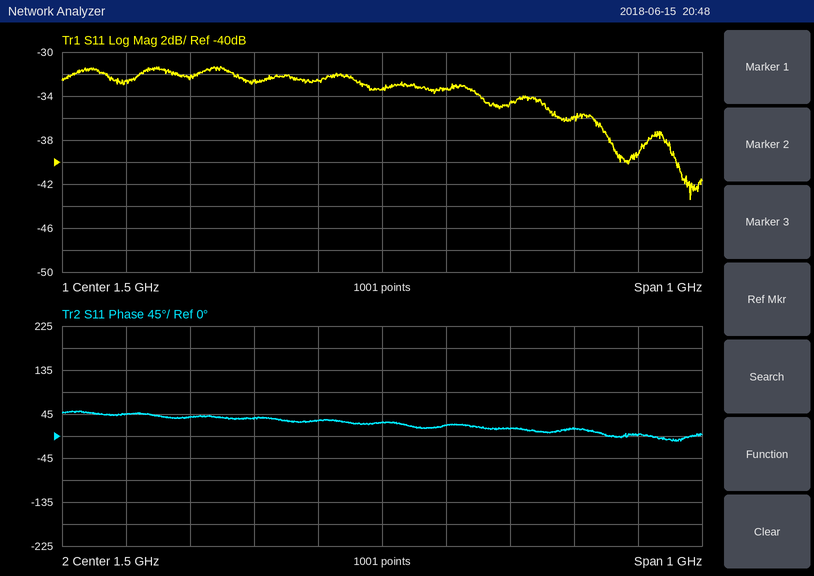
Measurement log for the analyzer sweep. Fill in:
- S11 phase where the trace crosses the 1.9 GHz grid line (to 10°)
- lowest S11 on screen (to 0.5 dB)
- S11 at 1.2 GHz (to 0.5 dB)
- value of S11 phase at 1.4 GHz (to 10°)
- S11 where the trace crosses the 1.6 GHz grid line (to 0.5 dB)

0°
-43.5 dB
-32.5 dB
30°
-33.5 dB
